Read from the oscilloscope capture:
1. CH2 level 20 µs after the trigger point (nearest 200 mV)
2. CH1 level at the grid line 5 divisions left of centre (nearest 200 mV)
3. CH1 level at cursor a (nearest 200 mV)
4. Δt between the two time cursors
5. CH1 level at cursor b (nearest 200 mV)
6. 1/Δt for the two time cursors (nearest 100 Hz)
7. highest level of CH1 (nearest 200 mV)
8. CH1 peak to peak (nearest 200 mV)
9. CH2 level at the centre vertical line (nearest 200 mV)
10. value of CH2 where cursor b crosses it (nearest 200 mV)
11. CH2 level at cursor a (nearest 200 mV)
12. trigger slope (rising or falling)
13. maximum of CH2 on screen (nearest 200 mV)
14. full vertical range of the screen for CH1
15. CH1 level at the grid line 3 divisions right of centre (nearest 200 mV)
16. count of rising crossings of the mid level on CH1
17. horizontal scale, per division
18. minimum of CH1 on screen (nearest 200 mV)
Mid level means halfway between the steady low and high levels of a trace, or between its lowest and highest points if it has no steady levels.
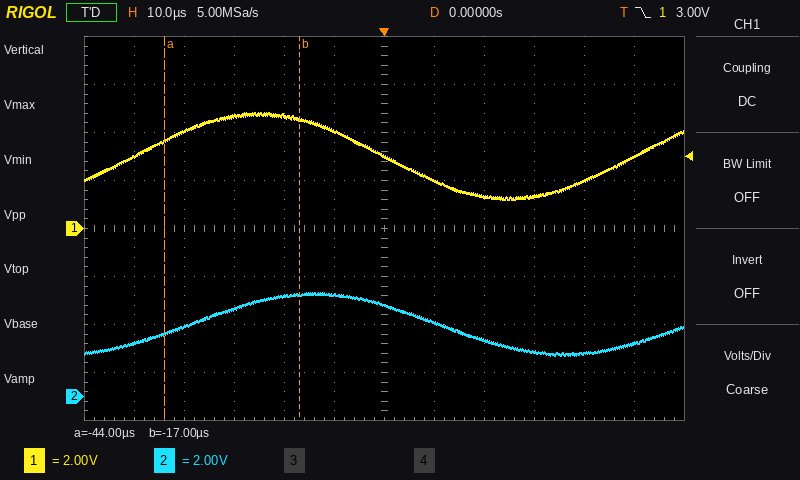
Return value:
2.4 V
3.0 V
3.6 V
27 µs
4.6 V
37.0 kHz
4.8 V
3.6 V
3.8 V
4.2 V
2.6 V
falling
4.4 V
16 V
1.4 V
2
10 µs
1.2 V
